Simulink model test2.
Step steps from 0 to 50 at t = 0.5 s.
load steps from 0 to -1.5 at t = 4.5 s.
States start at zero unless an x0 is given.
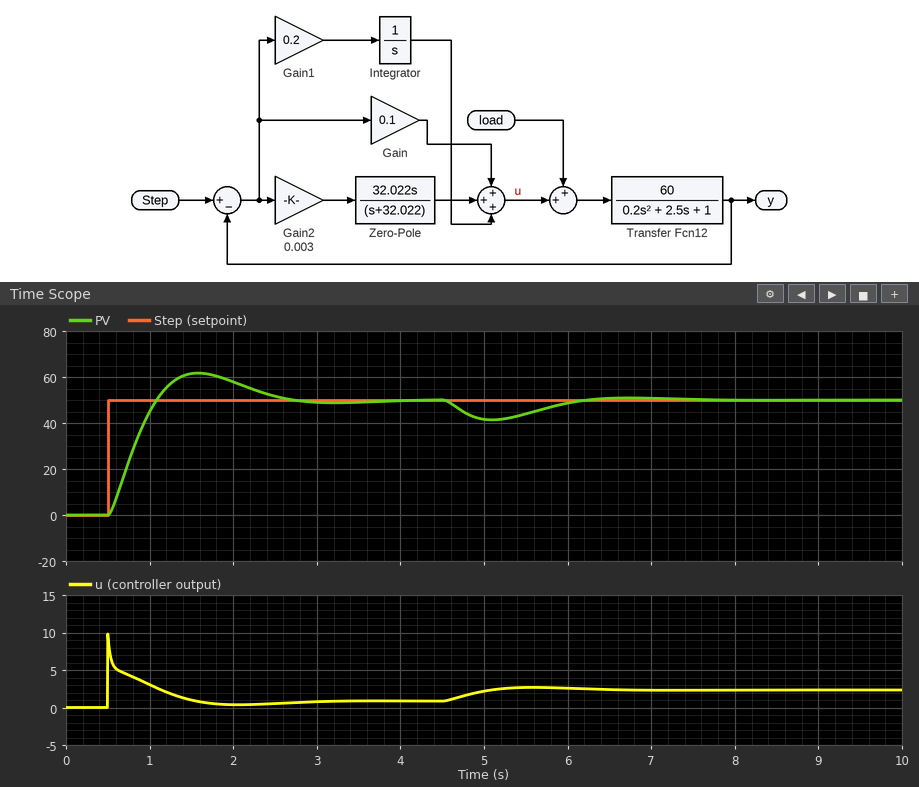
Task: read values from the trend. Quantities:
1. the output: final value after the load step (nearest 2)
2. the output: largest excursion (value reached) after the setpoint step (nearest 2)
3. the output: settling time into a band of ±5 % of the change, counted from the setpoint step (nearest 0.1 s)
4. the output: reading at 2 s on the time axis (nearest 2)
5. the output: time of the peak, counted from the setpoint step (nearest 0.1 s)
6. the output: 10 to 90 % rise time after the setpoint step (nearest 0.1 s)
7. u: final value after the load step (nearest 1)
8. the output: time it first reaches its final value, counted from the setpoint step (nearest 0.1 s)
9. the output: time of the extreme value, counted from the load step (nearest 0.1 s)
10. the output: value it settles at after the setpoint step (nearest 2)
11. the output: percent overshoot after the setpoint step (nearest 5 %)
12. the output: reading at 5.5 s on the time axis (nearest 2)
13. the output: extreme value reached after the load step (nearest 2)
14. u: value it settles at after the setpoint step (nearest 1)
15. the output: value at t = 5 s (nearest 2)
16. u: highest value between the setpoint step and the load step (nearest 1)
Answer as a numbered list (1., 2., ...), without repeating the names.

1. 50
2. 62
3. 1.9 s
4. 58
5. 1.1 s
6. 0.4 s
7. 2
8. 0.6 s
9. 0.6 s
10. 50
11. 25 %
12. 44
13. 42
14. 1
15. 42
16. 10
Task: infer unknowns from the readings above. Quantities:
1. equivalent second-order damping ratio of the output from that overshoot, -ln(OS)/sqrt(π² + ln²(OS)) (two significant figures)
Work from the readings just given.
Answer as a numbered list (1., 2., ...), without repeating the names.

1. 0.40
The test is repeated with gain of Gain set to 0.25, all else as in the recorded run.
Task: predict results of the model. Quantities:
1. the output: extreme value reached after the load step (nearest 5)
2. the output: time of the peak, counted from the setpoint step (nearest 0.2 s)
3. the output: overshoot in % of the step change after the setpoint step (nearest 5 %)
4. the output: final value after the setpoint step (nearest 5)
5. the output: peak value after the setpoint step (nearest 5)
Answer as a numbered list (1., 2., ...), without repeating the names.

1. 45
2. 0.6 s
3. 10 %
4. 50
5. 55
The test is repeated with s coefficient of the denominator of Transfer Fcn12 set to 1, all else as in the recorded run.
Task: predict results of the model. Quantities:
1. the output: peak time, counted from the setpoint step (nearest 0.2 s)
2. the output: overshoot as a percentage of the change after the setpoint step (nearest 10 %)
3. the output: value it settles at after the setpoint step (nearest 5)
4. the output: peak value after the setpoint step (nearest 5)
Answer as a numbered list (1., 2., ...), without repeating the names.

1. 0.6 s
2. 30 %
3. 50
4. 65
